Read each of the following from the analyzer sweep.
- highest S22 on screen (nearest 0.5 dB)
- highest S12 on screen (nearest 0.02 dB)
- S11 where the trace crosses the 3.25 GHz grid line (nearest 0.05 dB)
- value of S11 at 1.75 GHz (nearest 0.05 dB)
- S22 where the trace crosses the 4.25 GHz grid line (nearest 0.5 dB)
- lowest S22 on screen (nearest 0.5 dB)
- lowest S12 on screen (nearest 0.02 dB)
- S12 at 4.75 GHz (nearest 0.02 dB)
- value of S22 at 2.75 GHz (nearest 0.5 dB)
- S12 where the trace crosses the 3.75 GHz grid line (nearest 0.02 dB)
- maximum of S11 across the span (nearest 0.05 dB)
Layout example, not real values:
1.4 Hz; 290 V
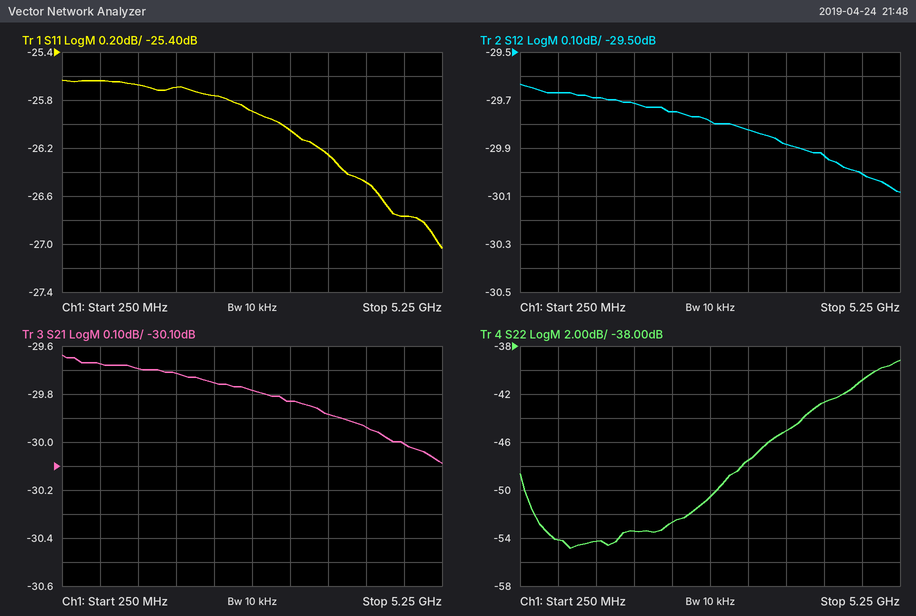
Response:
-39.0 dB; -29.64 dB; -26.05 dB; -25.70 dB; -42.5 dB; -55.0 dB; -30.08 dB; -30.00 dB; -50.5 dB; -29.88 dB; -25.65 dB
